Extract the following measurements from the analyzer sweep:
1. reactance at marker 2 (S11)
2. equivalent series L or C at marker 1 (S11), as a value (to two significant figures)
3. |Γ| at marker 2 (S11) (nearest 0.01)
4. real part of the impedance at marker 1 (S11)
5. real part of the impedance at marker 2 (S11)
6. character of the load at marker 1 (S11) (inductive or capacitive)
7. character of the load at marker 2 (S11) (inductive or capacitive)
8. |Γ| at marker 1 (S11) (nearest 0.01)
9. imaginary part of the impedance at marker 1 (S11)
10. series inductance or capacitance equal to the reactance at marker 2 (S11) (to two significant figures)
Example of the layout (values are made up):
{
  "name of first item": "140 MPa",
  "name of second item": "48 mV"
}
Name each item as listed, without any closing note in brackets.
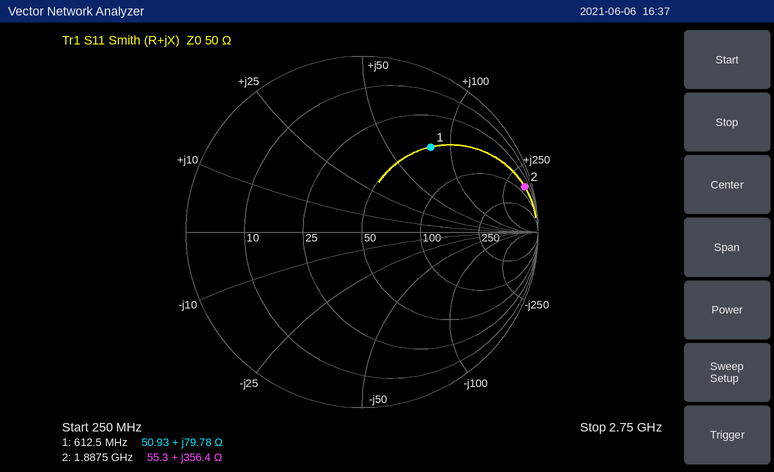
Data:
{
  "reactance at marker 2": "+356.4 Ω",
  "equivalent series L or C at marker 1 (S11), as a value": "21 nH",
  "|Γ| at marker 2 (S11)": "0.96",
  "real part of the impedance at marker 1": "50.93 Ω",
  "real part of the impedance at marker 2": "55.3 Ω",
  "character of the load at marker 1 (S11)": "inductive",
  "character of the load at marker 2 (S11)": "inductive",
  "|Γ| at marker 1 (S11)": "0.62",
  "imaginary part of the impedance at marker 1": "+79.78 Ω",
  "series inductance or capacitance equal to the reactance at marker 2 (S11)": "30 nH"
}
